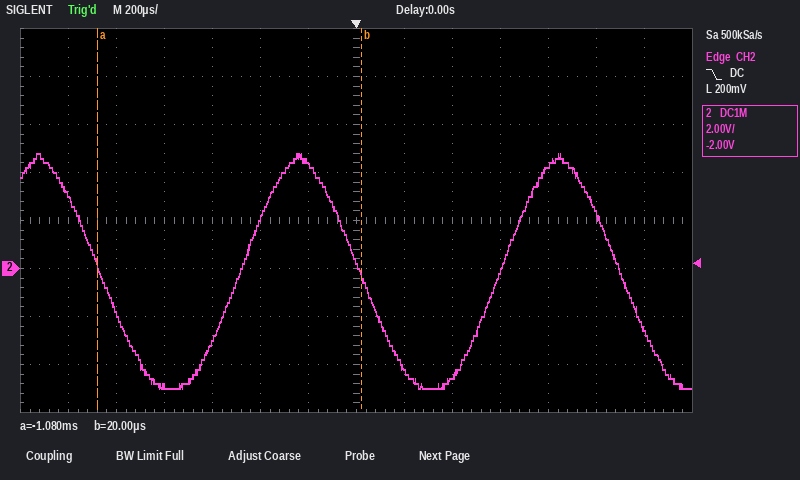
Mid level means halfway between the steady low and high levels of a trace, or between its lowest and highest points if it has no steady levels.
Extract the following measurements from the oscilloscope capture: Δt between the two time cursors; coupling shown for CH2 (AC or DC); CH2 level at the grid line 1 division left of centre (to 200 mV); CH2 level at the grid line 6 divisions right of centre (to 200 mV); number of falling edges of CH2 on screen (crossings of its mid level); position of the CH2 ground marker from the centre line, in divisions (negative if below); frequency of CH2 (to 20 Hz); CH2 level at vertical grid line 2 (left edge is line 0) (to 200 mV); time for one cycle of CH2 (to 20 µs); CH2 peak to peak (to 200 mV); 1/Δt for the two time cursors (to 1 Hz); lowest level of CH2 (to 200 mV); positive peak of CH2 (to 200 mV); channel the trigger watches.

1.10 ms
DC
4.4 V
-2.6 V
3
-1.0 div
920 Hz
-1.8 V
1.08 ms
9.8 V
909 Hz
-5.0 V
4.8 V
CH2
